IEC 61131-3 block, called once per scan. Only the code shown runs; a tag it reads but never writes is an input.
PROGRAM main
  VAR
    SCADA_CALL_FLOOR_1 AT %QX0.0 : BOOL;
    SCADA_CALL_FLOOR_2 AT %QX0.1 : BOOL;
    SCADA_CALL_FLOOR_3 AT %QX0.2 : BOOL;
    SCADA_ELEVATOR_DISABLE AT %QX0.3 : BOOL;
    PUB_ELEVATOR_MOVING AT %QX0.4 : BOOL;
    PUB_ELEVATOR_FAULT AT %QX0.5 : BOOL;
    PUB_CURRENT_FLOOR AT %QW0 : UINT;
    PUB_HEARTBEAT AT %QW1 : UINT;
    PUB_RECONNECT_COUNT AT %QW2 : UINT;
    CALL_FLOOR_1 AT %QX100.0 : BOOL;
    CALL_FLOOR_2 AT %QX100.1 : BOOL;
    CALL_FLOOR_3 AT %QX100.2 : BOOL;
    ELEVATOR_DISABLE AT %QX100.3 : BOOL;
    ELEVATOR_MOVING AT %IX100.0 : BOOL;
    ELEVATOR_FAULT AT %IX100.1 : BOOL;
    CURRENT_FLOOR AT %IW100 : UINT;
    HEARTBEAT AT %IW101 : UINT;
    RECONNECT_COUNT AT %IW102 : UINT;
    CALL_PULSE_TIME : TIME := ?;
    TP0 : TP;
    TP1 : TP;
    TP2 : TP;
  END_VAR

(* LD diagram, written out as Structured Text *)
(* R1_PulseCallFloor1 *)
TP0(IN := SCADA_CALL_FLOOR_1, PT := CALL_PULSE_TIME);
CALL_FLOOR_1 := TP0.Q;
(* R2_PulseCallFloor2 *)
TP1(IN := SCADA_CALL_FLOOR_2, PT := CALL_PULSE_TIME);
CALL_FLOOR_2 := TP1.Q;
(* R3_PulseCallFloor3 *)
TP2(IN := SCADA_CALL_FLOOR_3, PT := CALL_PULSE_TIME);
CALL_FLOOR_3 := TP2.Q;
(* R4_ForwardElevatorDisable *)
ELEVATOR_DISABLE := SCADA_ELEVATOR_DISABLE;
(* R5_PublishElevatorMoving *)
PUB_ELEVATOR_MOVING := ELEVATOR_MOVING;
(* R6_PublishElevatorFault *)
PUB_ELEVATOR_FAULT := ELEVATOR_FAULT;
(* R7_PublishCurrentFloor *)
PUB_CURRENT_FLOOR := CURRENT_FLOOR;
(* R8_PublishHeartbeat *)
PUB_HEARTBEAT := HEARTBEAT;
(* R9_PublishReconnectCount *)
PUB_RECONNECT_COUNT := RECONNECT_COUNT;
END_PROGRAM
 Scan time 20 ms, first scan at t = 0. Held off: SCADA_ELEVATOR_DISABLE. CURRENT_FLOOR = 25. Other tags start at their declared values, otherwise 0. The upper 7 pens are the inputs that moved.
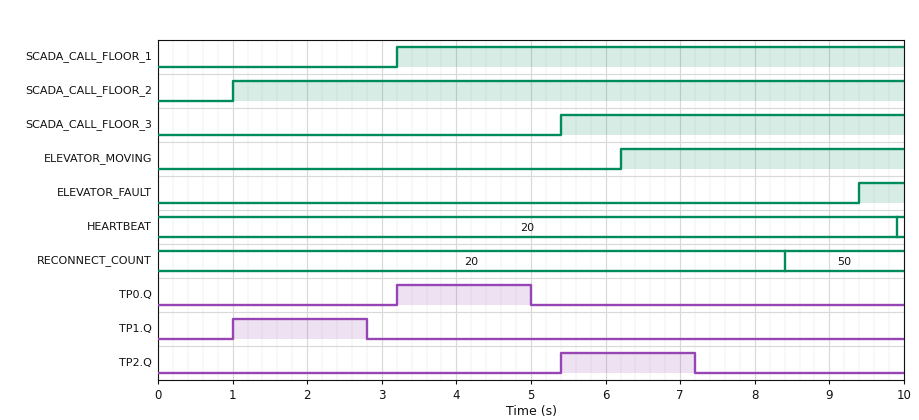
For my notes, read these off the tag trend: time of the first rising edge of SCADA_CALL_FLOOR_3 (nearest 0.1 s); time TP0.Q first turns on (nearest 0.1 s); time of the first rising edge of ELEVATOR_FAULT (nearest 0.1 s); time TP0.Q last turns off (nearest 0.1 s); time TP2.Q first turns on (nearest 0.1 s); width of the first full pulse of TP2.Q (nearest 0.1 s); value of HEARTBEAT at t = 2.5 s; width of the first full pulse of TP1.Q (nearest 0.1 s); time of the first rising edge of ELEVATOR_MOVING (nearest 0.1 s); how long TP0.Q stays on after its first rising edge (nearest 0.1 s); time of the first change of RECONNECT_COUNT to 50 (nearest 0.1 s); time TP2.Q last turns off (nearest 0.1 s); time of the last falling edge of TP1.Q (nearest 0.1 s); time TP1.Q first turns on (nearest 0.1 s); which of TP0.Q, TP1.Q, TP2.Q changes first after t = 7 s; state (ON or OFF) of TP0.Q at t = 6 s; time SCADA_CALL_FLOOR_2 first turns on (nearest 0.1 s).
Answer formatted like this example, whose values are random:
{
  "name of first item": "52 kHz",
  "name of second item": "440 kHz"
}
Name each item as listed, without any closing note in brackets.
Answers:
{
  "time of the first rising edge of SCADA_CALL_FLOOR_3": "5.4 s",
  "time TP0.Q first turns on": "3.2 s",
  "time of the first rising edge of ELEVATOR_FAULT": "9.4 s",
  "time TP0.Q last turns off": "5.0 s",
  "time TP2.Q first turns on": "5.4 s",
  "width of the first full pulse of TP2.Q": "1.8 s",
  "value of HEARTBEAT at t = 2.5 s": "20",
  "width of the first full pulse of TP1.Q": "1.8 s",
  "time of the first rising edge of ELEVATOR_MOVING": "6.2 s",
  "how long TP0.Q stays on after its first rising edge": "1.8 s",
  "time of the first change of RECONNECT_COUNT to 50": "8.4 s",
  "time TP2.Q last turns off": "7.2 s",
  "time of the last falling edge of TP1.Q": "2.8 s",
  "time TP1.Q first turns on": "1.0 s",
  "which of TP0.Q, TP1.Q, TP2.Q changes first after t = 7 s": "TP2.Q",
  "state (ON or OFF) of TP0.Q at t = 6 s": "OFF",
  "time SCADA_CALL_FLOOR_2 first turns on": "1.0 s"
}
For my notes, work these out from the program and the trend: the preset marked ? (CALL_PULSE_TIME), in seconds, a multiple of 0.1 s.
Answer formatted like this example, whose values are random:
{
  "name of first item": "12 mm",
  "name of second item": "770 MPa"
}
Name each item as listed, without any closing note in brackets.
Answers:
{
  "the preset marked ? (CALL_PULSE_TIME), in seconds, a multiple of 0.1 s": "1.8 s"
}
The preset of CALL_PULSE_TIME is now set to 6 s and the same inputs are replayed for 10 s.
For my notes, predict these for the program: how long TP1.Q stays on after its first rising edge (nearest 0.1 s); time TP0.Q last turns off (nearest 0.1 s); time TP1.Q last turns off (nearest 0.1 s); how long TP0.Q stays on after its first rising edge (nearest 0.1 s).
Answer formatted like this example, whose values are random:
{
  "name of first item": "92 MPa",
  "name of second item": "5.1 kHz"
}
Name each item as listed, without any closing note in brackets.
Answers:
{
  "how long TP1.Q stays on after its first rising edge": "6.0 s",
  "time TP0.Q last turns off": "9.2 s",
  "time TP1.Q last turns off": "7.0 s",
  "how long TP0.Q stays on after its first rising edge": "6.0 s"
}
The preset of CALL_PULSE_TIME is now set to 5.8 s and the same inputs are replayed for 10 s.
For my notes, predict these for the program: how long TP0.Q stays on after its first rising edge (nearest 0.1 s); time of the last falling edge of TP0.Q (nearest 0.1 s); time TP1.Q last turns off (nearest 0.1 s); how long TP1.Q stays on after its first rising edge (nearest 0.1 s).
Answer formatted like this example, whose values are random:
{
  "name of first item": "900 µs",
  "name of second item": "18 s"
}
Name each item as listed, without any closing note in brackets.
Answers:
{
  "how long TP0.Q stays on after its first rising edge": "5.8 s",
  "time of the last falling edge of TP0.Q": "9.0 s",
  "time TP1.Q last turns off": "6.8 s",
  "how long TP1.Q stays on after its first rising edge": "5.8 s"
}
